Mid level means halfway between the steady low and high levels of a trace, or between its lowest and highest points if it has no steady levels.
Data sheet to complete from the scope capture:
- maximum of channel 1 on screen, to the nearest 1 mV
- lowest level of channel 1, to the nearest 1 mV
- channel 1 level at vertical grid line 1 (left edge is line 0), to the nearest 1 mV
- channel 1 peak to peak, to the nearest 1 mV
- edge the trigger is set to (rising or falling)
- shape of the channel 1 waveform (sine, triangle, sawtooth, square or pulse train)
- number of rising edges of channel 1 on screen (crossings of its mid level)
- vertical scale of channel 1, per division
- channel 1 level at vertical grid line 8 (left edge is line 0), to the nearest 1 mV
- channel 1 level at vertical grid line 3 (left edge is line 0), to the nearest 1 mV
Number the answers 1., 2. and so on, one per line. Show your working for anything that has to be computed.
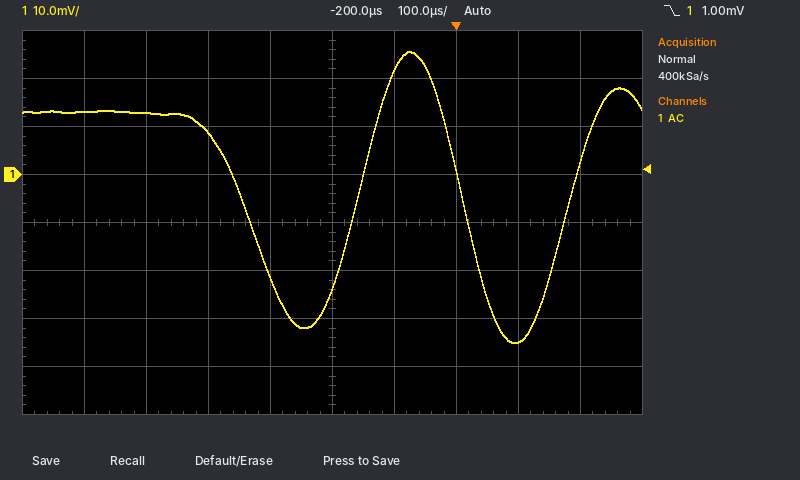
1. 26 mV
2. -35 mV
3. 13 mV
4. 26 mV − (-35 mV) = 61 mV
5. falling
6. sine
7. 2
8. 10 mV
9. -35 mV
10. 9 mV
